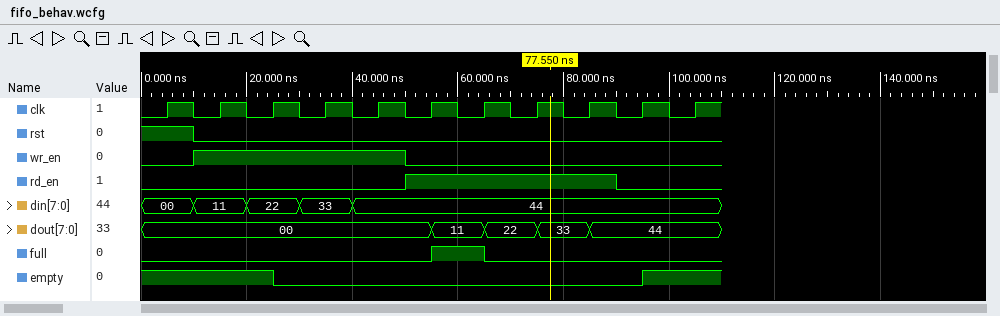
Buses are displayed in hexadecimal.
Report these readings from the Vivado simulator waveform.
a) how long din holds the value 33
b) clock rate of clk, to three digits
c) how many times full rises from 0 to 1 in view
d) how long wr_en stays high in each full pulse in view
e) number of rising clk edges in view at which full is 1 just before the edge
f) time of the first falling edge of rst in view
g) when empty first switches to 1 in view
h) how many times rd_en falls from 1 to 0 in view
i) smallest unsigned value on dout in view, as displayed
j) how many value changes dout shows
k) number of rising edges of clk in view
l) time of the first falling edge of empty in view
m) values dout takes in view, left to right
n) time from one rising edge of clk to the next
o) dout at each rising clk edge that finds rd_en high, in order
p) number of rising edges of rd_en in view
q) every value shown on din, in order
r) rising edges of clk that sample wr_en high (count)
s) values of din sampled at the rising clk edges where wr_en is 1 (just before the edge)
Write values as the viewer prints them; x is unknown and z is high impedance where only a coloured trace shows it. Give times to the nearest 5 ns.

10 ns
100 MHz
1
40 ns
1
10 ns
95 ns
1
00
4
11
25 ns
00, 11, 22, 33, 44
10 ns
00, 11, 22, 33
1
00, 11, 22, 33, 44
4
11, 22, 33, 44
